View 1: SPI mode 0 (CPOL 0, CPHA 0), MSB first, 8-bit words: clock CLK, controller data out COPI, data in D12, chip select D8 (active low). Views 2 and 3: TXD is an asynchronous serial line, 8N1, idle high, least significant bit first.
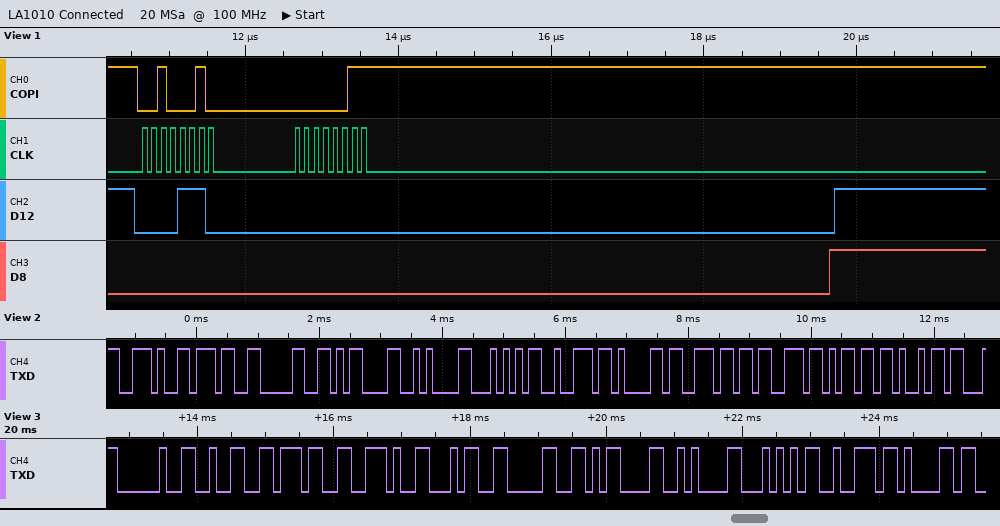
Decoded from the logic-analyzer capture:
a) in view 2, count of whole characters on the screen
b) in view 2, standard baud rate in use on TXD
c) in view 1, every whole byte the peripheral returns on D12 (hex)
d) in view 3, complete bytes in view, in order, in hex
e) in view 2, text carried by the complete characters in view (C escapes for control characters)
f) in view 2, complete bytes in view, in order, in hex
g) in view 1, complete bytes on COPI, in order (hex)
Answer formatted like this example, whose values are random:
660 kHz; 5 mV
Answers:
12; 9600 baud; 0x0E 0x00; 0x20 0x32 0x37 0x2E 0x34 0x30 0x0D 0x0A 0x54 0x72 0x61; ".70\r\nTransmi"; 2E 37 30 0D 0A 54 72 61 6E 73 6D 69; 0x22 0x03
